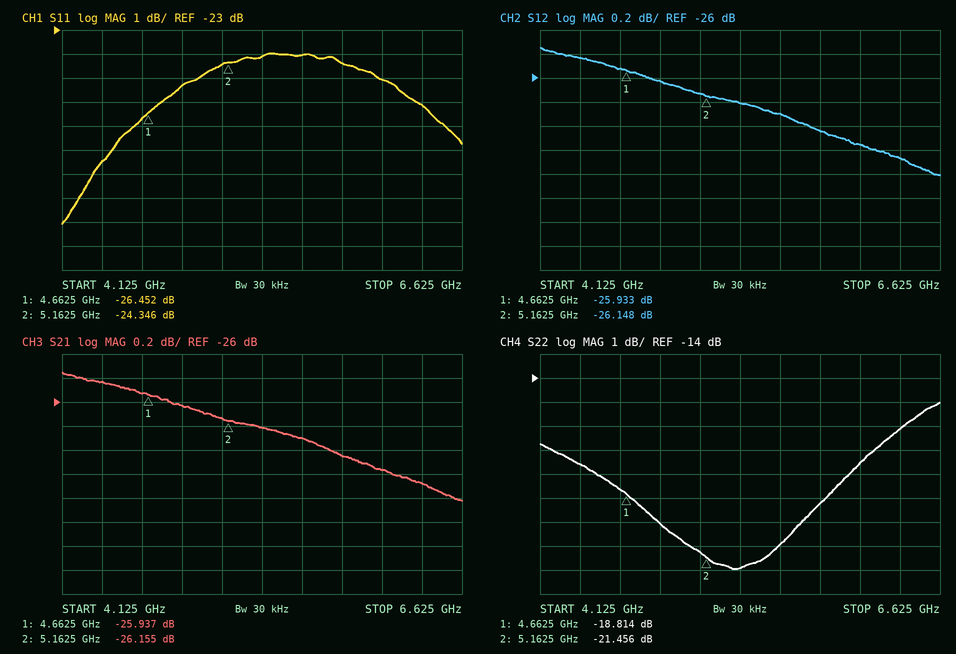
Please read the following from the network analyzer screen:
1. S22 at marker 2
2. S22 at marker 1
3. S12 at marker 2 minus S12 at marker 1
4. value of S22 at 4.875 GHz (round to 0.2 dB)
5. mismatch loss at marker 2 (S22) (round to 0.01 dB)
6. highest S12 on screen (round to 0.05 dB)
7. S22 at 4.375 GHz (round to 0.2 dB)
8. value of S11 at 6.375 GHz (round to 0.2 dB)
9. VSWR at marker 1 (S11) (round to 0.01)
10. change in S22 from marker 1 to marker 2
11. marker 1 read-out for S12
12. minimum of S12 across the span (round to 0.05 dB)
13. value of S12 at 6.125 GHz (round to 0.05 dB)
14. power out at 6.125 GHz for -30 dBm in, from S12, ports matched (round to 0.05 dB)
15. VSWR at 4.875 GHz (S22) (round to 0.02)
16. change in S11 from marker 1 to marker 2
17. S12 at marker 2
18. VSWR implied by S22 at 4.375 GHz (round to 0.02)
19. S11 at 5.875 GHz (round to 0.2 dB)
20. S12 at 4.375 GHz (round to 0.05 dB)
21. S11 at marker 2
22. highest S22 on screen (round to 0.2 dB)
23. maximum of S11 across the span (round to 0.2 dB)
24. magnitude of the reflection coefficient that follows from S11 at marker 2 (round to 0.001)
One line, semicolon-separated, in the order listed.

-21.456 dB; -18.814 dB; -0.215 dB; -20.0 dB; 0.03 dB; -25.75 dB; -17.6 dB; -26.2 dB; 1.10; -2.642 dB; -25.933 dB; -26.80 dB; -26.55 dB; -56.55 dBm; 1.22; 2.106 dB; -26.148 dB; 1.30; -24.4 dB; -25.85 dB; -24.346 dB; -15.0 dB; -24.0 dB; 0.061
